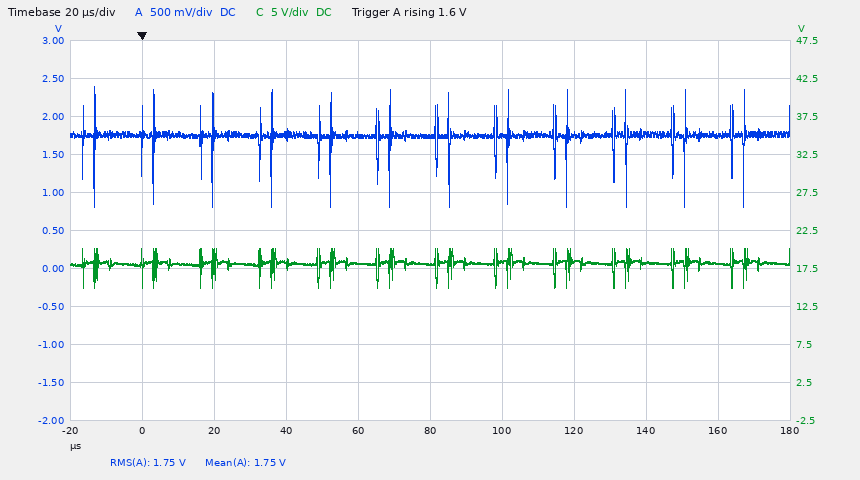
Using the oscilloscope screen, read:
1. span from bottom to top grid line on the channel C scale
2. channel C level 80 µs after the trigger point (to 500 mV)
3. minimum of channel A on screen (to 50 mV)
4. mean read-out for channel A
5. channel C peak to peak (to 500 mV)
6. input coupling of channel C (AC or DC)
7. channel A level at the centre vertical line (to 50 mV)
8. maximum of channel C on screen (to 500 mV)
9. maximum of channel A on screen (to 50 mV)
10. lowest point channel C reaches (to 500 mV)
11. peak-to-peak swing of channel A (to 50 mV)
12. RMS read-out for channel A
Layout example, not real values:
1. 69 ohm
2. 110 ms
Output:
1. 50 V
2. 18.0 V
3. 800 mV
4. 1.75 V
5. 5.0 V
6. DC
7. 1.75 V
8. 20.0 V
9. 2.40 V
10. 15.0 V
11. 1.60 V
12. 1.75 V
